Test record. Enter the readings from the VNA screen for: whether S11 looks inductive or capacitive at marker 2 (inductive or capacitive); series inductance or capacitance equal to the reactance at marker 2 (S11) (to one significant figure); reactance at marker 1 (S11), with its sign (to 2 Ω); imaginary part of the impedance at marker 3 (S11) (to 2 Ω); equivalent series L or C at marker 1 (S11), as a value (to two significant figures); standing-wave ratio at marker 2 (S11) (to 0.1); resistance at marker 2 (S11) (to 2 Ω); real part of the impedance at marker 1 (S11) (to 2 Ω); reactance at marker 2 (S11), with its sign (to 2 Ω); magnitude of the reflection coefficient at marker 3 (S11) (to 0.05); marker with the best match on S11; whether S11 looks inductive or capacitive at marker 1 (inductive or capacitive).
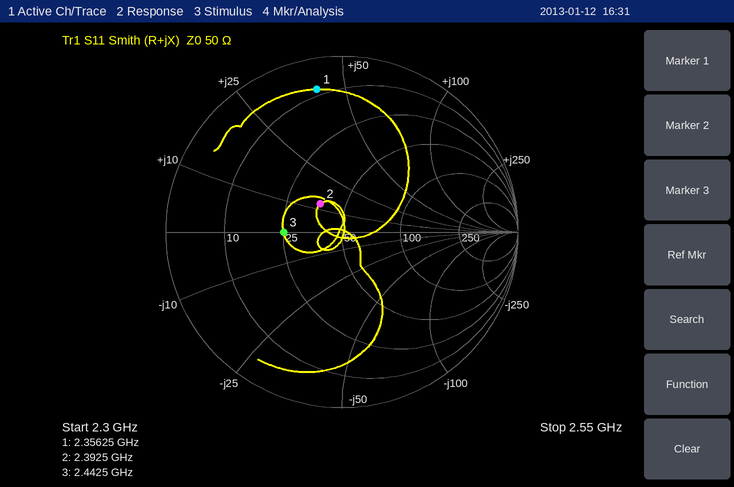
inductive
800 pH
+42 Ω
0 Ω
2.8 nH
1.5
38 Ω
8 Ω
+12 Ω
0.35
marker 2
inductive
